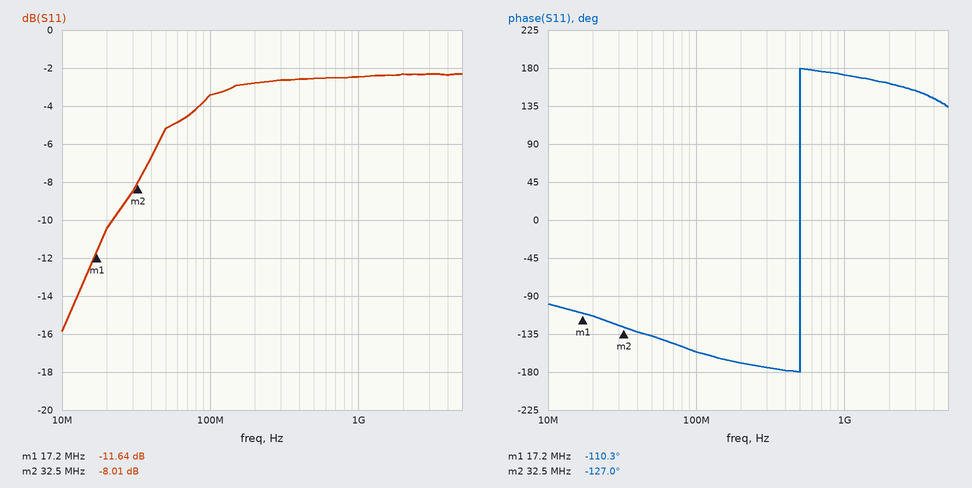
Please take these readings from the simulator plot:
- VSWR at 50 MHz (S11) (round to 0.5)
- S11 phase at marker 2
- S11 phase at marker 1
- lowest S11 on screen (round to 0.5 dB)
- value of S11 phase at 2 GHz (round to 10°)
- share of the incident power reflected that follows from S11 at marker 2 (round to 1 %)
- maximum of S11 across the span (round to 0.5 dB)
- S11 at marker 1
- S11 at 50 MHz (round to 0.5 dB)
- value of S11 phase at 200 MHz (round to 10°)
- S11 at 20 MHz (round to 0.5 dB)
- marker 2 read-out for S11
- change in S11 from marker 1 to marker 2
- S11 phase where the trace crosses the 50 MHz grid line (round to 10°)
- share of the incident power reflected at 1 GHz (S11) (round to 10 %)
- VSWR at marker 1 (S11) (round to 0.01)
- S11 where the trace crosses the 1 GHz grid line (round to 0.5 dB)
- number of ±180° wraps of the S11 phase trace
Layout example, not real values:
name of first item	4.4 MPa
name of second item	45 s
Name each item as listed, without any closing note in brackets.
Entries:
VSWR at 50 MHz (S11)	3.5
S11 phase at marker 2	-127.0°
S11 phase at marker 1	-110.3°
lowest S11 on screen	-16.0 dB
value of S11 phase at 2 GHz	160°
share of the incident power reflected that follows from S11 at marker 2	16 %
maximum of S11 across the span	-2.5 dB
S11 at marker 1	-11.64 dB
S11 at 50 MHz	-5.0 dB
value of S11 phase at 200 MHz	-170°
S11 at 20 MHz	-10.5 dB
marker 2 read-out for S11	-8.01 dB
change in S11 from marker 1 to marker 2	3.63 dB
S11 phase where the trace crosses the 50 MHz grid line	-140°
share of the incident power reflected at 1 GHz (S11)	60 %
VSWR at marker 1 (S11)	1.71
S11 where the trace crosses the 1 GHz grid line	-2.5 dB
number of ±180° wraps of the S11 phase trace	1
